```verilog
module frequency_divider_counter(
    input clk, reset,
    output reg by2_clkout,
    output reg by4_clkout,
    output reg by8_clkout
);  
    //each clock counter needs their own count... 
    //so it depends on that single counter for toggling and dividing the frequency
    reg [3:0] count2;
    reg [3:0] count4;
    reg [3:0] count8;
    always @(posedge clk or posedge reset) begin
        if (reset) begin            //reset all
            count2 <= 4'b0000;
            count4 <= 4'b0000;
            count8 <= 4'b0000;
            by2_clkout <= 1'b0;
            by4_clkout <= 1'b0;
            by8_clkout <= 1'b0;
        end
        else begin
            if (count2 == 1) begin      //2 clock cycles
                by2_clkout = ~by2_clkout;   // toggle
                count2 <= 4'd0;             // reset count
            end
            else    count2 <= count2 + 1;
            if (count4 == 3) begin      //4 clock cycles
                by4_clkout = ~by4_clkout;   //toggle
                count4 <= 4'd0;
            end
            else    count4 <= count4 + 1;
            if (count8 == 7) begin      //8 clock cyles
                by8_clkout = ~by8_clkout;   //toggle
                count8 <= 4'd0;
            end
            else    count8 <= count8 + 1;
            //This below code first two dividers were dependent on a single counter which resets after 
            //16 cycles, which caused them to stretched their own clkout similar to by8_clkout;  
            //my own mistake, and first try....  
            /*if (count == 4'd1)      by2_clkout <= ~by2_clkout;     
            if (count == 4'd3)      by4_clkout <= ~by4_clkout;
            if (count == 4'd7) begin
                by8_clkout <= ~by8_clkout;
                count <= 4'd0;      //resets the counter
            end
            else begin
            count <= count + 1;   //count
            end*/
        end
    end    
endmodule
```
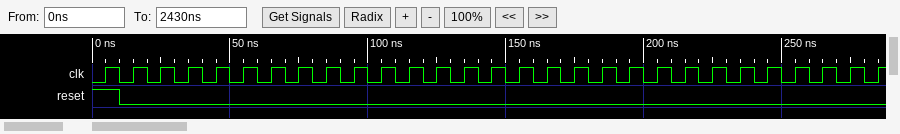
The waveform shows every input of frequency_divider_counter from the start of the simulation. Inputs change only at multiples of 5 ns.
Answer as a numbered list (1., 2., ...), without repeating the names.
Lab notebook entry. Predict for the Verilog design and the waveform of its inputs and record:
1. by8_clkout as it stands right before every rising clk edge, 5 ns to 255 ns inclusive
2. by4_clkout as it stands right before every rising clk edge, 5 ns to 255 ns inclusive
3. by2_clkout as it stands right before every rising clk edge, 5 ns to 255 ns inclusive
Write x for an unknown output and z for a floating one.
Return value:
1. 0 0 0 0 0 0 0 0 0 1 1 1 1 1 1 1 1 0 0 0 0 0 0 0 0 1
2. 0 0 0 0 0 1 1 1 1 0 0 0 0 1 1 1 1 0 0 0 0 1 1 1 1 0
3. 0 0 0 1 1 0 0 1 1 0 0 1 1 0 0 1 1 0 0 1 1 0 0 1 1 0
